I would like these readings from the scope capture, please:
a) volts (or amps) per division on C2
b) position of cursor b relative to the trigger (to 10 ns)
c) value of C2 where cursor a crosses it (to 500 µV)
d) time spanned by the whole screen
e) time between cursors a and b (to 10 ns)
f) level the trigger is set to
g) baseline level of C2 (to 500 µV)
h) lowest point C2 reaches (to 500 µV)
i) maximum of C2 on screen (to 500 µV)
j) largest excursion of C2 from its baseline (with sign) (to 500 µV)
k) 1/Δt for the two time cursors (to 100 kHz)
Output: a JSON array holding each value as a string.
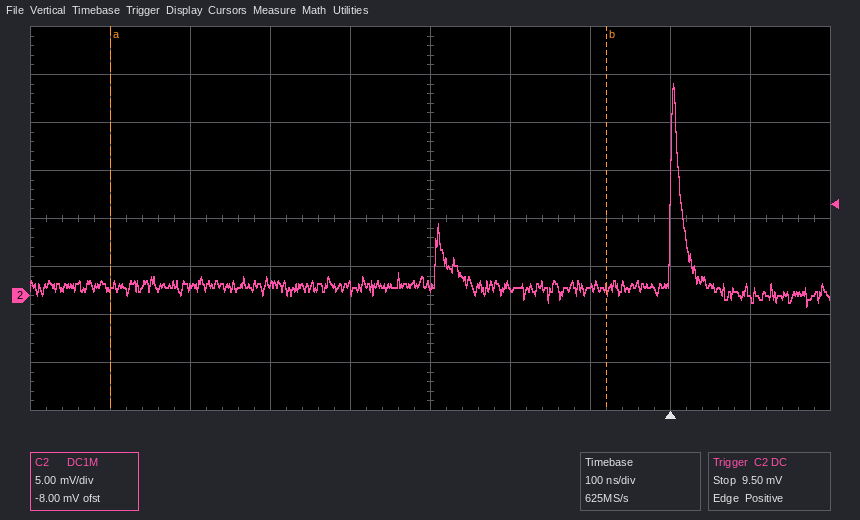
["5 mV", "-80 ns", "1.0 mV", "1 µs", "620 ns", "9.50 mV", "1.0 mV", "-1.0 mV", "22.0 mV", "+21.0 mV", "1.6 MHz"]
